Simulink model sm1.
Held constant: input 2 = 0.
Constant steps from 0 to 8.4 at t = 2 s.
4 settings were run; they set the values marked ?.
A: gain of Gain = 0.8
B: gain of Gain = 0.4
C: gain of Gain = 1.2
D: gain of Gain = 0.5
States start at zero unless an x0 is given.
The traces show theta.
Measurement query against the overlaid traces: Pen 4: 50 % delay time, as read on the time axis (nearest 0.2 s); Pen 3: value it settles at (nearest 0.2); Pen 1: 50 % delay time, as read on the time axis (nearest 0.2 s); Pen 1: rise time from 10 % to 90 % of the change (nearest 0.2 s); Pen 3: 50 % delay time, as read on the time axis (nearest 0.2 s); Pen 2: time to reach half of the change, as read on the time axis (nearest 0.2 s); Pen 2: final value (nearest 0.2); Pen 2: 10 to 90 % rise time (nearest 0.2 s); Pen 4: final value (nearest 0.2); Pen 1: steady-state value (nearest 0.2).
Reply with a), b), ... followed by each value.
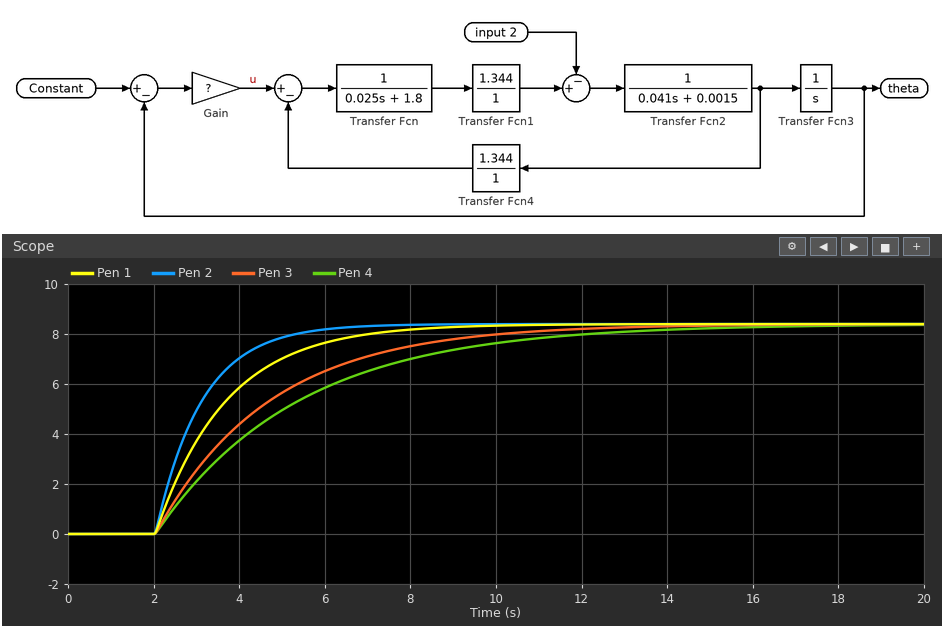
a) 4.4 s
b) 8.4
c) 3.2 s
d) 3.6 s
e) 3.8 s
f) 2.8 s
g) 8.4
h) 2.4 s
i) 8.4
j) 8.4
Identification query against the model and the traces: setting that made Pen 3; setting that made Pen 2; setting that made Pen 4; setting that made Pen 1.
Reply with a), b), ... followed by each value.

a) D
b) C
c) B
d) A
